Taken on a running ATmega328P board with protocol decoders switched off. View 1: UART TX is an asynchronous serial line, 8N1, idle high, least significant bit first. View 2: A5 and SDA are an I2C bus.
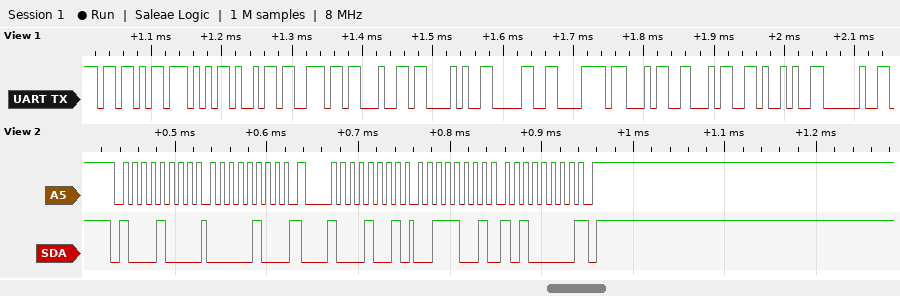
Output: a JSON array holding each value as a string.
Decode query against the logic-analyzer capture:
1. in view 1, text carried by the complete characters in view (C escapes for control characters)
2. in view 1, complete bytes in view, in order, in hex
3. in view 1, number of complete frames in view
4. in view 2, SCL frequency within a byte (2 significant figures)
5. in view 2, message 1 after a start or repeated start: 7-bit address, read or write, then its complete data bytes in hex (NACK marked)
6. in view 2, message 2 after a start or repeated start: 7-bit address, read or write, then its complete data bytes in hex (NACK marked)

["\"[Wind(0x44) \"", "5B 57 69 6E 64 28 30 78 34 34 29 20", "12", "100 kHz", "0x44 write: 04", "0x44 read: 39 A0 NACK"]
